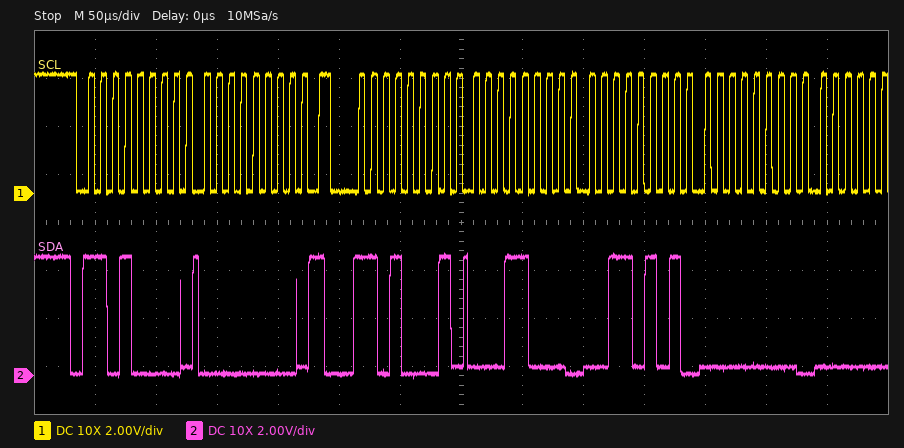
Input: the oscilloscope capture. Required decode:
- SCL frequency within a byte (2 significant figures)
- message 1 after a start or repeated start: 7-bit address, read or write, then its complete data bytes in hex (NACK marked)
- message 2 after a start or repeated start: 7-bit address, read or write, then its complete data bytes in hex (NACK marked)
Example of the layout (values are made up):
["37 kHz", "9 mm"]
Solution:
["100 kHz", "0x68 write: 00", "0x68 read: 18 35 00"]
